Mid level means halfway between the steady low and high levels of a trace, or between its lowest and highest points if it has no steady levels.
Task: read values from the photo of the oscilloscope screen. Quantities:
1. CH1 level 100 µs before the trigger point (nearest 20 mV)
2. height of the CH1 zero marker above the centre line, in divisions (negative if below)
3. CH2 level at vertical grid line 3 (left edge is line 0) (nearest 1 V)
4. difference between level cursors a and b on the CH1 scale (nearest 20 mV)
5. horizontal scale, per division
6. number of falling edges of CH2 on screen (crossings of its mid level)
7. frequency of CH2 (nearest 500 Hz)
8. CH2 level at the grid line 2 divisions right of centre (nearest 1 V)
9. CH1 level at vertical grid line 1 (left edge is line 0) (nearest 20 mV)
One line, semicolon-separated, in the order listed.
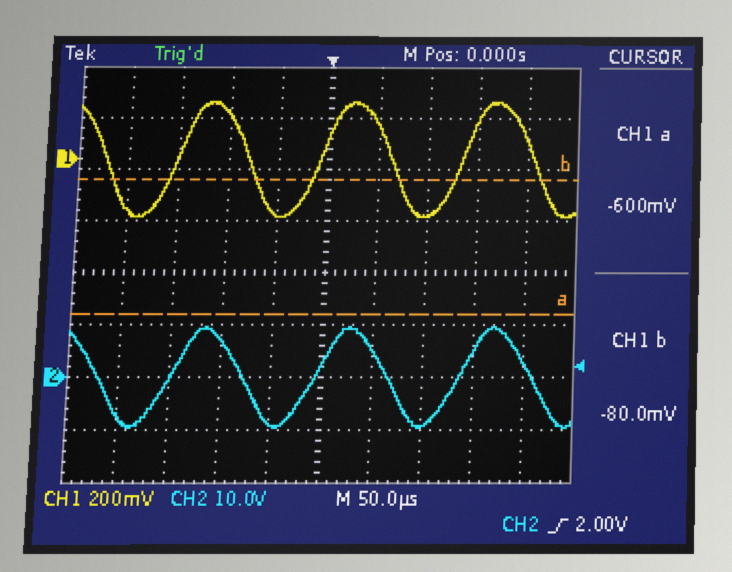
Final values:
180 mV; +2.2 div; 7 V; 520 mV; 50 µs; 4; 7.0 kHz; -9 V; -200 mV
